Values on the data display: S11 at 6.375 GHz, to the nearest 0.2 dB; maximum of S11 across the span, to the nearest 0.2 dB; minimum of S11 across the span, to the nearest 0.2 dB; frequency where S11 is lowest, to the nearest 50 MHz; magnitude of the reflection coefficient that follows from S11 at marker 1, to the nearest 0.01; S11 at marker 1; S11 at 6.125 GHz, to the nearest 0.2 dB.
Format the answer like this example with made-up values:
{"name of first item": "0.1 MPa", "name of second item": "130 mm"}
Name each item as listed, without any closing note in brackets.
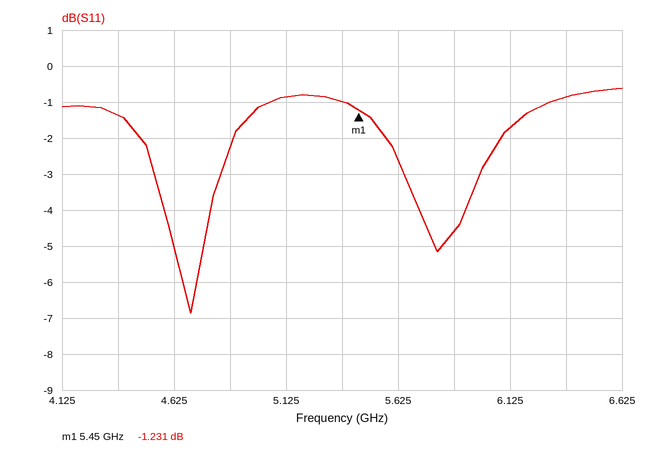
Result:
{"S11 at 6.375 GHz, to the nearest 0.2 dB": "-0.8 dB", "maximum of S11 across the span, to the nearest 0.2 dB": "-0.6 dB", "minimum of S11 across the span, to the nearest 0.2 dB": "-6.8 dB", "frequency where S11 is lowest, to the nearest 50 MHz": "4.70 GHz", "magnitude of the reflection coefficient that follows from S11 at marker 1, to the nearest 0.01": "0.87", "S11 at marker 1": "-1.231 dB", "S11 at 6.125 GHz, to the nearest 0.2 dB": "-1.8 dB"}
